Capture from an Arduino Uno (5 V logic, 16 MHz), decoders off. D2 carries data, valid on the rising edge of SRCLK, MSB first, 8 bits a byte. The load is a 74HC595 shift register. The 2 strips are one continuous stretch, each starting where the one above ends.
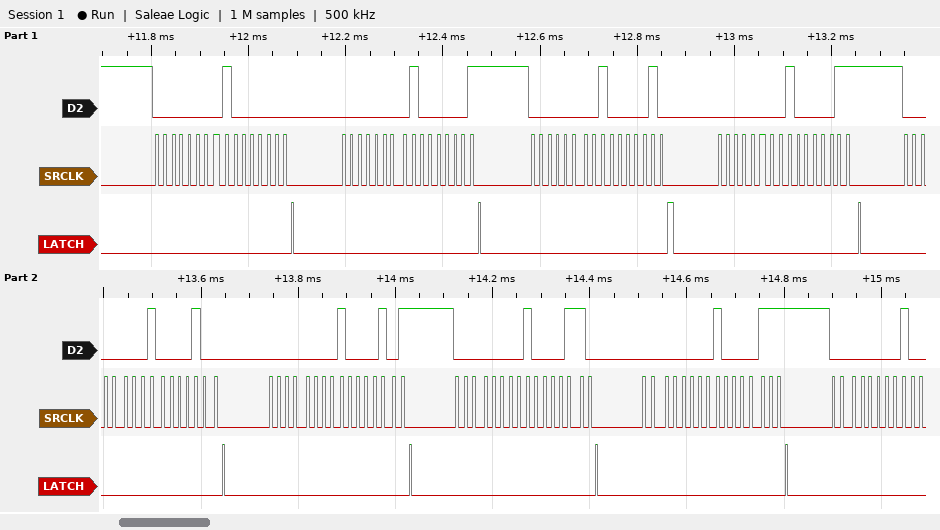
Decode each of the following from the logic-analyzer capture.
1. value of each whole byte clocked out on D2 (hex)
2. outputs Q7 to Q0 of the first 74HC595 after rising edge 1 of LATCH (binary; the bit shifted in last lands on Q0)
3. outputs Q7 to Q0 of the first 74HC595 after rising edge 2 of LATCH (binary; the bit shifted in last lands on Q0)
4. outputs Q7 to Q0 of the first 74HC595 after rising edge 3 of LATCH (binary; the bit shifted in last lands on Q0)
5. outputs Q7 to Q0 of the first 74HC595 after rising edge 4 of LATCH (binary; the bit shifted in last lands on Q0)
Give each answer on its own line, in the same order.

00 80 00 81 00 82 00 83 00 84 00 85 00 86 00 87 00
10000000
10000001
10000010
10000011
